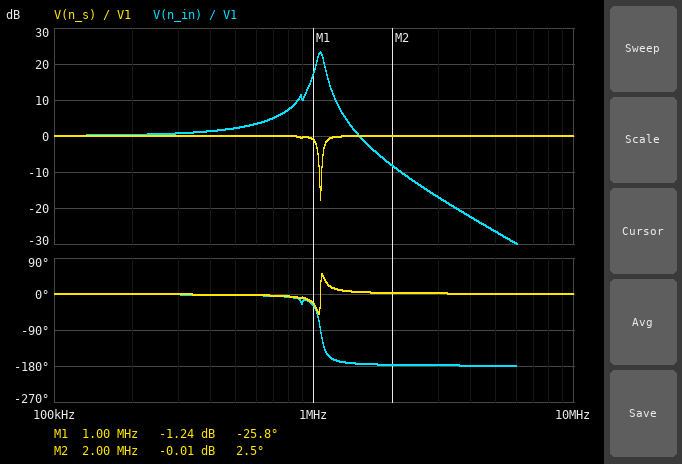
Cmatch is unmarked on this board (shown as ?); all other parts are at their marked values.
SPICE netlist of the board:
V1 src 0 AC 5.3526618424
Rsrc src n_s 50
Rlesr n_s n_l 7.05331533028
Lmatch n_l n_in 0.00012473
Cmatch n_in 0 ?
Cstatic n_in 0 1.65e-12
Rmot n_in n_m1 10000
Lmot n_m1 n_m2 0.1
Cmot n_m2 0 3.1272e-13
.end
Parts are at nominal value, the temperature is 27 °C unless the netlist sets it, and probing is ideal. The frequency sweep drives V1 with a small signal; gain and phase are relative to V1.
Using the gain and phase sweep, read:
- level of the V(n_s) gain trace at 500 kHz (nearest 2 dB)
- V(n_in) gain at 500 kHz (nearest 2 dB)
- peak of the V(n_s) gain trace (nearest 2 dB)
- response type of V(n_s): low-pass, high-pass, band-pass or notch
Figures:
0 dB
2 dB
0 dB
notch
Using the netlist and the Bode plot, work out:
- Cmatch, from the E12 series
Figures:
180 pF
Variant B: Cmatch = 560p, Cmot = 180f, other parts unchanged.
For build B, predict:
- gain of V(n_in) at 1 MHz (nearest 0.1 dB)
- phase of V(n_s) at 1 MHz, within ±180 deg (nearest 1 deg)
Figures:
-5.0 dB
6 deg
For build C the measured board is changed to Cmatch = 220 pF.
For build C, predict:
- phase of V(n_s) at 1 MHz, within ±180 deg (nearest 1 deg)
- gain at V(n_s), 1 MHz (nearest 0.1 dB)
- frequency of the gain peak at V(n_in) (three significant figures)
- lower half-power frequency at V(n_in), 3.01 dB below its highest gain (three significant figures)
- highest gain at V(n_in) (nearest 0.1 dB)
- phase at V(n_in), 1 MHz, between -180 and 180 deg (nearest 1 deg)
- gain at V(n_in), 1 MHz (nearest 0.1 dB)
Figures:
36 deg
-2.7 dB
961 kHz
929 kHz
22.3 dB
-137 deg
18.7 dB
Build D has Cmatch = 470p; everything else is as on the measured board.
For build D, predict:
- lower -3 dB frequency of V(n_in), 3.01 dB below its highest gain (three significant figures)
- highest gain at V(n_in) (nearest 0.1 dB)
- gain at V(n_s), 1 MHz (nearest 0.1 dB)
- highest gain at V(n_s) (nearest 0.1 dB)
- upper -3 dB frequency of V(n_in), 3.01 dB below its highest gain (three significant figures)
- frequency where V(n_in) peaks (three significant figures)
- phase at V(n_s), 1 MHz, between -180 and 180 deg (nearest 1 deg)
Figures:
616 kHz
19.1 dB
-0.1 dB
0 dB
689 kHz
654 kHz
6 deg
